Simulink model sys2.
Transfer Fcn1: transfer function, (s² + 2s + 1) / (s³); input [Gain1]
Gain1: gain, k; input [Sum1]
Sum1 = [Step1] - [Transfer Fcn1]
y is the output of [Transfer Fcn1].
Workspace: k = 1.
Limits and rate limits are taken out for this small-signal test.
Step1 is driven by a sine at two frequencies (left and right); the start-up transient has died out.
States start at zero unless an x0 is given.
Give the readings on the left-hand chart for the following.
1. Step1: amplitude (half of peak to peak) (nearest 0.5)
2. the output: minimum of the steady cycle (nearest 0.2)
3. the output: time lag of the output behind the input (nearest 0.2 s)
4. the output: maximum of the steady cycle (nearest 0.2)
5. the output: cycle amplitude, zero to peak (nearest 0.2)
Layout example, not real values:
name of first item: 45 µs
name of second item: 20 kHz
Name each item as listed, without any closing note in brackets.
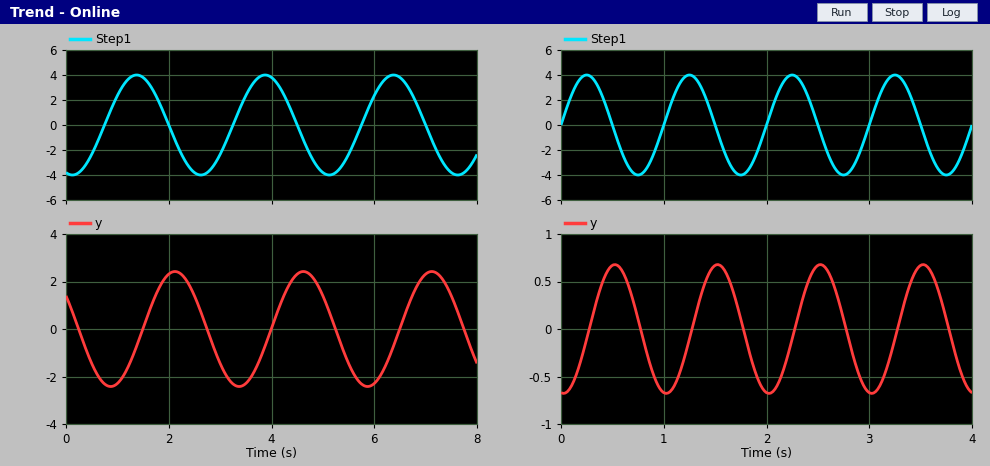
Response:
Step1: amplitude (half of peak to peak): 4.0
the output: minimum of the steady cycle: -2.4
the output: time lag of the output behind the input: 0.8 s
the output: maximum of the steady cycle: 2.4
the output: cycle amplitude, zero to peak: 2.4
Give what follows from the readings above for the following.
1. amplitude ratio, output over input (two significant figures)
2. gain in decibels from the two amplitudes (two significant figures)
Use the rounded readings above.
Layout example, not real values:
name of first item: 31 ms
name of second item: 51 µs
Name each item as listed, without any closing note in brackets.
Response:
amplitude ratio, output over input: 0.60
gain in decibels from the two amplitudes: -4.4 dB
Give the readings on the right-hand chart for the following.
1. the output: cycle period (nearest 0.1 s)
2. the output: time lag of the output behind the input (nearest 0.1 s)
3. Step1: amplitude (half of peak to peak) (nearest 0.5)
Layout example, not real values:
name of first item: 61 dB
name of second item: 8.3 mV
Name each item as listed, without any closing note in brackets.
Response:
the output: cycle period: 1.0 s
the output: time lag of the output behind the input: 0.3 s
Step1: amplitude (half of peak to peak): 4.0
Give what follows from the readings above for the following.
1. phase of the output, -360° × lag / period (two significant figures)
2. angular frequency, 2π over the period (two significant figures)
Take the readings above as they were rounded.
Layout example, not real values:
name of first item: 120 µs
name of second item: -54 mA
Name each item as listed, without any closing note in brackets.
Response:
phase of the output, -360° × lag / period: -110°
angular frequency, 2π over the period: 6.3 rad/s
